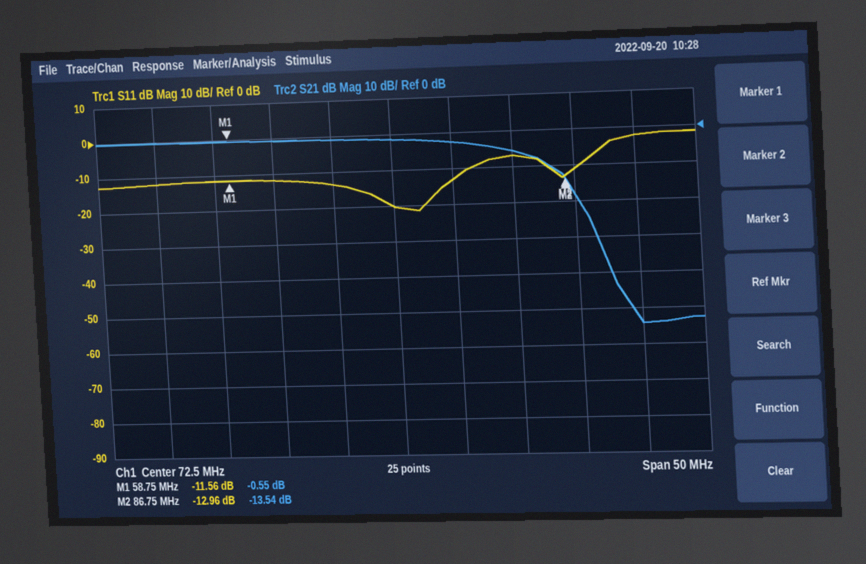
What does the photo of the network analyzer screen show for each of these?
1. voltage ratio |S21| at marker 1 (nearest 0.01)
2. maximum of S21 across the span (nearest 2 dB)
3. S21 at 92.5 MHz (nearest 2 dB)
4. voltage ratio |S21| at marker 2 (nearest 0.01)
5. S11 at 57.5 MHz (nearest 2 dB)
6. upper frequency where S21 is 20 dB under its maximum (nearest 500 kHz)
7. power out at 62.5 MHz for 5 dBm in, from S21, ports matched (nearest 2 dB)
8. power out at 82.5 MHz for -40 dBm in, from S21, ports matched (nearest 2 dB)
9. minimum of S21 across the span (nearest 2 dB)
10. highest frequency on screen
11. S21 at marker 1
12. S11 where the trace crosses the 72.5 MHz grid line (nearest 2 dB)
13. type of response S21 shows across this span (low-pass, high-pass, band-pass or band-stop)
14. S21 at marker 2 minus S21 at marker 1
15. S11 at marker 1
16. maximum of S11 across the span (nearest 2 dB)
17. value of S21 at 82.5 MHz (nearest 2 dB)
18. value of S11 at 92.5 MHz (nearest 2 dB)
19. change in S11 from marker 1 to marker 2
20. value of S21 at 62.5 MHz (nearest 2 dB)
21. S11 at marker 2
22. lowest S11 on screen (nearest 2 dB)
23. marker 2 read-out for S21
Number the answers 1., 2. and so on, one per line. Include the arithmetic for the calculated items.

1. 10^(-0.55/20) ≈ 0.94
2. 0 dB
3. -54 dB
4. 10^(-13.54/20) ≈ 0.21
5. -12 dB
6. 88.0 MHz
7. 5 dBm + (0 dB) = 4 dBm
8. -40 dBm + (-6 dB) = -46 dBm
9. -54 dB
10. 97.5 MHz
11. -0.55 dB
12. -20 dB
13. low-pass
14. -13.54 − (-0.55) = -12.99 dB
15. -11.56 dB
16. -2 dB
17. -6 dB
18. -2 dB
19. -12.96 − (-11.56) = -1.40 dB
20. 0 dB
21. -12.96 dB
22. -22 dB
23. -13.54 dB
